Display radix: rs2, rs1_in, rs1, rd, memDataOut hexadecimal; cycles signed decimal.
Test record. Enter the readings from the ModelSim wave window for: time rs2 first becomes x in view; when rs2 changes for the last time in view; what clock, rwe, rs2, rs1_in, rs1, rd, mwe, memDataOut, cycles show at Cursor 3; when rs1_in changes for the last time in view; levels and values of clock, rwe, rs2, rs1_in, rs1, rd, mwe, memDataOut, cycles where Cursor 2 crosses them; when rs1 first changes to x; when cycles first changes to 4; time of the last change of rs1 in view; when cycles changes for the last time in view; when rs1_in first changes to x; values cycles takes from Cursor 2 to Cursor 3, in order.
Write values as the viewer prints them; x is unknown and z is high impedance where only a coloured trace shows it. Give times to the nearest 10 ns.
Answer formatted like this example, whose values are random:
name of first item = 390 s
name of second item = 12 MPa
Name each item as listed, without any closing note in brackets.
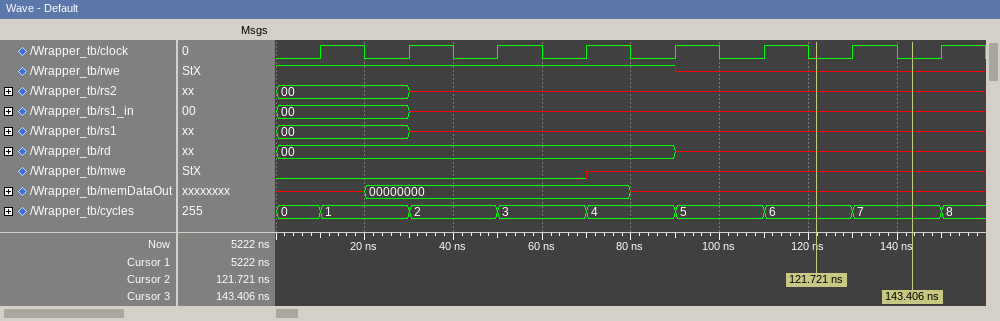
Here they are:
time rs2 first becomes x in view = 30 ns
when rs2 changes for the last time in view = 30 ns
what clock, rwe, rs2, rs1_in, rs1, rd, mwe, memDataOut, cycles show at Cursor 3 = clock=0, rwe=x, rs2=x, rs1_in=x, rs1=x, rd=x, mwe=x, memDataOut=x, cycles=7
when rs1_in changes for the last time in view = 30 ns
levels and values of clock, rwe, rs2, rs1_in, rs1, rd, mwe, memDataOut, cycles where Cursor 2 crosses them = clock=0, rwe=x, rs2=x, rs1_in=x, rs1=x, rd=x, mwe=x, memDataOut=x, cycles=6
when rs1 first changes to x = 30 ns
when cycles first changes to 4 = 70 ns
time of the last change of rs1 in view = 30 ns
when cycles changes for the last time in view = 150 ns
when rs1_in first changes to x = 30 ns
values cycles takes from Cursor 2 to Cursor 3, in order = 6, 7
